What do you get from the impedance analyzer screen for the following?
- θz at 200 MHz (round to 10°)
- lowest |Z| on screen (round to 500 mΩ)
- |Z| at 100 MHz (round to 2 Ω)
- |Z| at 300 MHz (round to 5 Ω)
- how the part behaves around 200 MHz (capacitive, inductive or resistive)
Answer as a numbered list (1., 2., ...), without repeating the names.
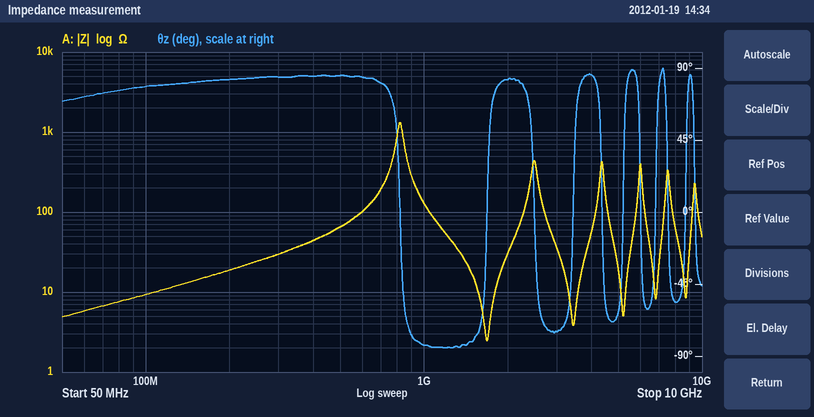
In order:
1. 80°
2. 2.5 Ω
3. 10 Ω
4. 30 Ω
5. inductive
